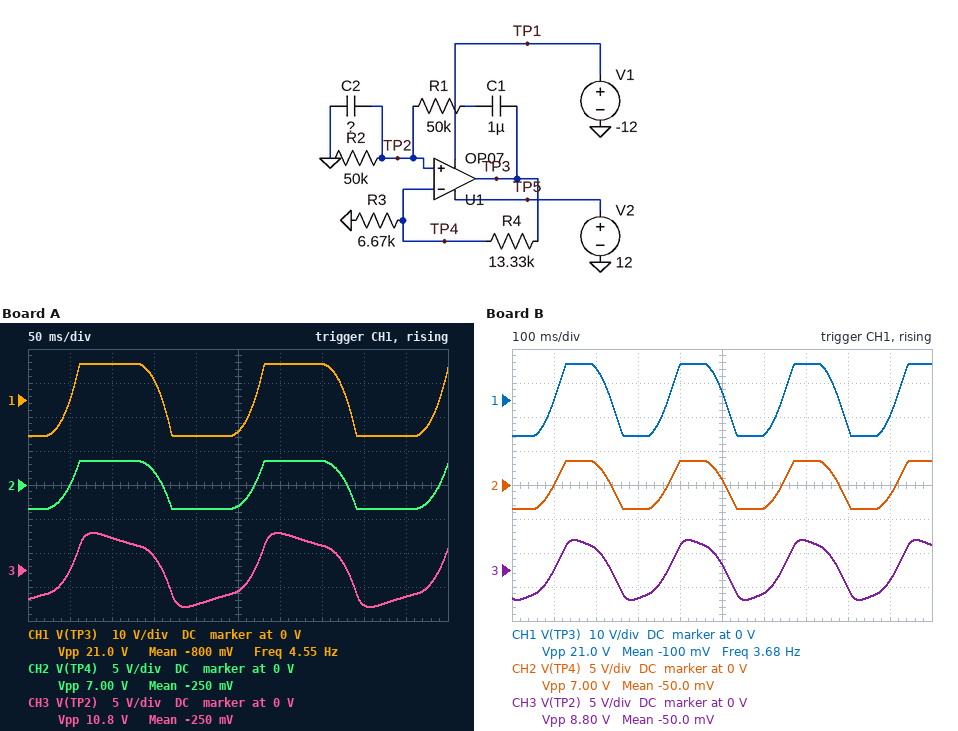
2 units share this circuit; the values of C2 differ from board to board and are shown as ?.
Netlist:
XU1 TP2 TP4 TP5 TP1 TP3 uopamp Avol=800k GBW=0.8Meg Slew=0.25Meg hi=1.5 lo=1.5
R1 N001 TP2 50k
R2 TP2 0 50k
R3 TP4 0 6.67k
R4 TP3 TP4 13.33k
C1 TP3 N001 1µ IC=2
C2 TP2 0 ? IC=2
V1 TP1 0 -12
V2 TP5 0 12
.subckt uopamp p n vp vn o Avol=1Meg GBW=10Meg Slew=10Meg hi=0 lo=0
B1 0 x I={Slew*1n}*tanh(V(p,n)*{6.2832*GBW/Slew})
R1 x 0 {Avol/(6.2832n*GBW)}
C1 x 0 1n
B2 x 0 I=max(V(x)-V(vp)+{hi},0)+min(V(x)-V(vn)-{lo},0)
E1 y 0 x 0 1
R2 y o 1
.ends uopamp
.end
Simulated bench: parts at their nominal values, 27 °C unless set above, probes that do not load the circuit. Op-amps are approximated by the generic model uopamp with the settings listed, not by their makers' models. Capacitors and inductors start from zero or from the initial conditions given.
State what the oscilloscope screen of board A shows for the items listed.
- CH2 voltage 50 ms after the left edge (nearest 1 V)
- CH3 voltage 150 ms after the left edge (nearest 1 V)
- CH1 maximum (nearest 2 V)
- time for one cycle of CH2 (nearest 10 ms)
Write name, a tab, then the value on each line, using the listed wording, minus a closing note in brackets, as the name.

CH2 voltage 50 ms after the left edge	0 V
CH3 voltage 150 ms after the left edge	2 V
CH1 maximum	10 V
time for one cycle of CH2	220 ms
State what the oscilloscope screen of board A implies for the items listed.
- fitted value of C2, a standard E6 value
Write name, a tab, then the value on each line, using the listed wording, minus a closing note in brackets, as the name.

fitted value of C2, a standard E6 value	330 nF
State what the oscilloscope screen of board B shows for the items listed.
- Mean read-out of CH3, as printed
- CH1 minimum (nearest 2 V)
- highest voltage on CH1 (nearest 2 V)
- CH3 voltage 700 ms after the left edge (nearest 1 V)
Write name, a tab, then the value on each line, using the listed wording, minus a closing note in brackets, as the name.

Mean read-out of CH3, as printed	-50.0 mV
CH1 minimum	-10 V
highest voltage on CH1	10 V
CH3 voltage 700 ms after the left edge	4 V
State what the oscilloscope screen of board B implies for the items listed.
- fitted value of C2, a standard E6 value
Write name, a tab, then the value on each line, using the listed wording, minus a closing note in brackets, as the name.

fitted value of C2, a standard E6 value	680 nF
